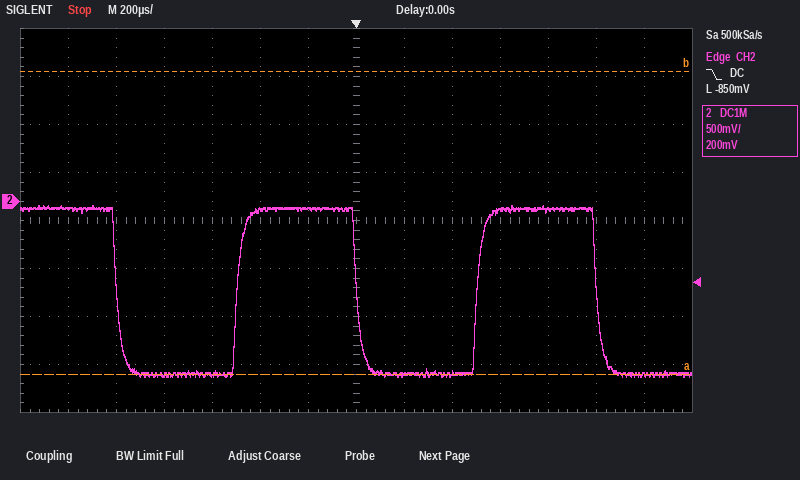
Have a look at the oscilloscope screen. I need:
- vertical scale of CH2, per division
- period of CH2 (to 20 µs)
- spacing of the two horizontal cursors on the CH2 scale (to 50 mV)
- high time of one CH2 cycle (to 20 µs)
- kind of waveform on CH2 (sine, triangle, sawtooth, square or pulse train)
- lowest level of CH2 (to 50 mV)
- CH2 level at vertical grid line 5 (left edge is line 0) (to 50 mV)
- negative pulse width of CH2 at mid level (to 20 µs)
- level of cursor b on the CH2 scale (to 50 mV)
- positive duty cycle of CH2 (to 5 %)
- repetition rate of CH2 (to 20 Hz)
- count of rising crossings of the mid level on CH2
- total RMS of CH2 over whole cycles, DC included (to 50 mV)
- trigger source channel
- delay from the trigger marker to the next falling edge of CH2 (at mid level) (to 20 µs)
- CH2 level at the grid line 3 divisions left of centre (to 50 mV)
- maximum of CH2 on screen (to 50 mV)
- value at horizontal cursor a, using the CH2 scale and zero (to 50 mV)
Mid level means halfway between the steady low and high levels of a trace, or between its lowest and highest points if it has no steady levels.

500 mV
1.00 ms
3.15 V
500 µs
square
-1.80 V
-100 mV
500 µs
1.35 V
50 %
1.00 kHz
2
1.25 V
CH2
1.00 ms
-1.80 V
-50 mV
-1.80 V
